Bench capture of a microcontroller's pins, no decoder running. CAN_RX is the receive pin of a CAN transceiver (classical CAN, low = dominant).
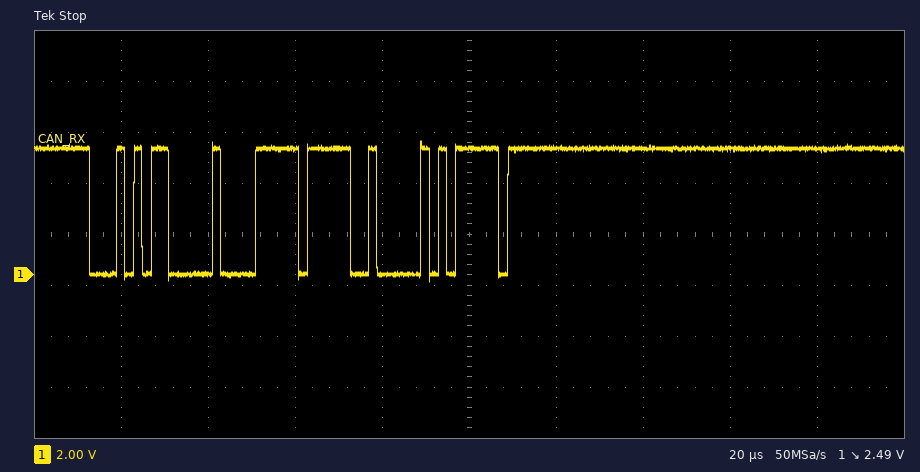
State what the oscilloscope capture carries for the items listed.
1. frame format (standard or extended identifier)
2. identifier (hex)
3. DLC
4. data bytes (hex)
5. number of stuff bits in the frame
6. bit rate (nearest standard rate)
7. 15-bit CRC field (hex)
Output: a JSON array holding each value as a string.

["standard", "0x158", "1", "FF", "4", "500 kbit/s", "0x502F"]
